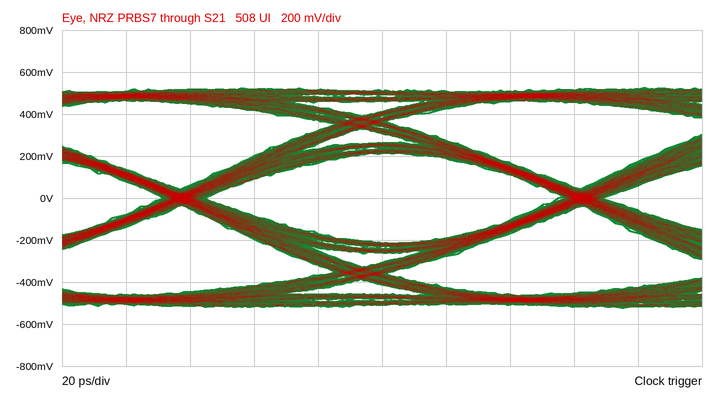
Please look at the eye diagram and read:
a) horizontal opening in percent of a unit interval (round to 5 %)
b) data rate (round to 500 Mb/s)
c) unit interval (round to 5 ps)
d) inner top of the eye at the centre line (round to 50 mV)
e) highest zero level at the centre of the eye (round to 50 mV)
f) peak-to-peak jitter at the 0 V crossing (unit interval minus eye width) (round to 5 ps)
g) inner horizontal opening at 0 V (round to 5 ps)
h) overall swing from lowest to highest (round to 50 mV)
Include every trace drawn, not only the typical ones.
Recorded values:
90 %
8.0 Gb/s
125 ps
200 mV
-200 mV
15 ps
110 ps
1.05 V
